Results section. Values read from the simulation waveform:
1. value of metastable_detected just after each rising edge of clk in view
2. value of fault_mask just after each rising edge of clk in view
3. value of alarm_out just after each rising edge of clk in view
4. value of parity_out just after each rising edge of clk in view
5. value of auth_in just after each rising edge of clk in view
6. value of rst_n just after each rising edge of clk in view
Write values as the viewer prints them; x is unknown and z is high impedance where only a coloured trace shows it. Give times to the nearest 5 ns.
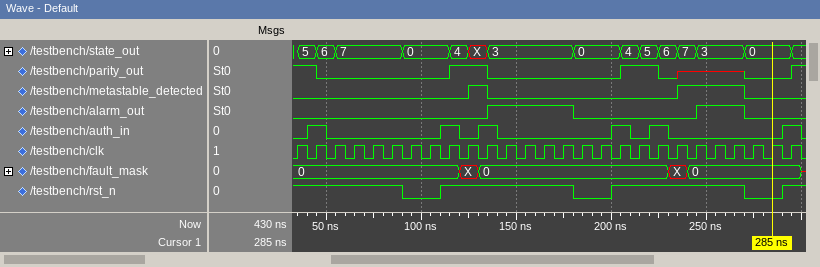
0 0 0 0 0 0 0 0 0 1 0 0 0 0 0 0 0 0 0 0 1 1 1 1 0 0 0
0, 0, 0, 0, 0, 0, 0, 0, 0, X, 0, 0, 0, 0, 0, 0, 0, 0, 0, 0, X, 0, 0, 0, 0, 0, 0
0 0 0 0 0 0 0 0 0 0 1 1 1 1 1 0 0 0 0 0 0 1 1 1 0 0 0
1 0 0 0 0 0 0 0 1 1 0 0 0 0 0 0 0 1 1 0 x x x x 0 0 1
0 1 0 0 0 0 0 0 1 0 1 0 0 0 0 0 0 1 0 1 0 0 0 0 0 0 1
1 1 1 1 1 1 0 0 1 1 1 1 1 1 1 0 0 1 1 1 1 1 1 1 0 0 1
